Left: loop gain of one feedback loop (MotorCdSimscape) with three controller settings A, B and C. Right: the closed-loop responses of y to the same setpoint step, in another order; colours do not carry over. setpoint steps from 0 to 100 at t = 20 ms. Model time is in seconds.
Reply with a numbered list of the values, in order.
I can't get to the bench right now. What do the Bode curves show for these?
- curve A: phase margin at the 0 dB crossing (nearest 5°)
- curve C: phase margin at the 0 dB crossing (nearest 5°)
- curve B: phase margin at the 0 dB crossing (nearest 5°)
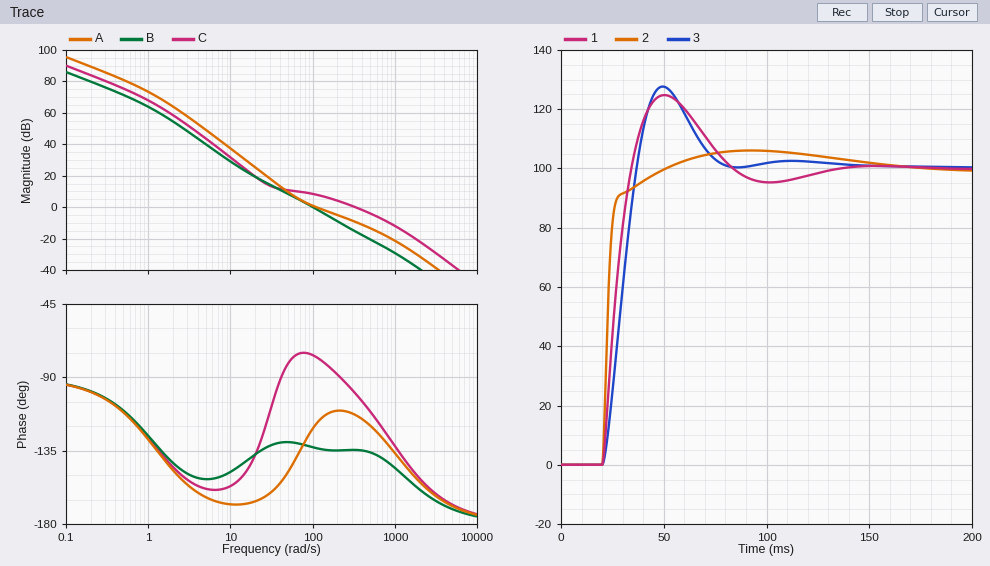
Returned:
1. 60°
2. 80°
3. 45°
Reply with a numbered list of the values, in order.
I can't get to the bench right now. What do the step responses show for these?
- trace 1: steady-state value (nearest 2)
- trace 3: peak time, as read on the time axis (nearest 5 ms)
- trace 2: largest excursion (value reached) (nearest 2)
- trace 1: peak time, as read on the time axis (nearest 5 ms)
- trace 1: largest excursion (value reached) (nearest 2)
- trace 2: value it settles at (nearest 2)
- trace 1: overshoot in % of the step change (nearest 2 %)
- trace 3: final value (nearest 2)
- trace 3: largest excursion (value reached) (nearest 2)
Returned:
1. 100
2. 50 ms
3. 106
4. 50 ms
5. 124
6. 100
7. 24 %
8. 100
9. 128
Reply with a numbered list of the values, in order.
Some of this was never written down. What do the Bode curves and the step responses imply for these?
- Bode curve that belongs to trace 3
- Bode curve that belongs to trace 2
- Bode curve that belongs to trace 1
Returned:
1. B
2. C
3. A
